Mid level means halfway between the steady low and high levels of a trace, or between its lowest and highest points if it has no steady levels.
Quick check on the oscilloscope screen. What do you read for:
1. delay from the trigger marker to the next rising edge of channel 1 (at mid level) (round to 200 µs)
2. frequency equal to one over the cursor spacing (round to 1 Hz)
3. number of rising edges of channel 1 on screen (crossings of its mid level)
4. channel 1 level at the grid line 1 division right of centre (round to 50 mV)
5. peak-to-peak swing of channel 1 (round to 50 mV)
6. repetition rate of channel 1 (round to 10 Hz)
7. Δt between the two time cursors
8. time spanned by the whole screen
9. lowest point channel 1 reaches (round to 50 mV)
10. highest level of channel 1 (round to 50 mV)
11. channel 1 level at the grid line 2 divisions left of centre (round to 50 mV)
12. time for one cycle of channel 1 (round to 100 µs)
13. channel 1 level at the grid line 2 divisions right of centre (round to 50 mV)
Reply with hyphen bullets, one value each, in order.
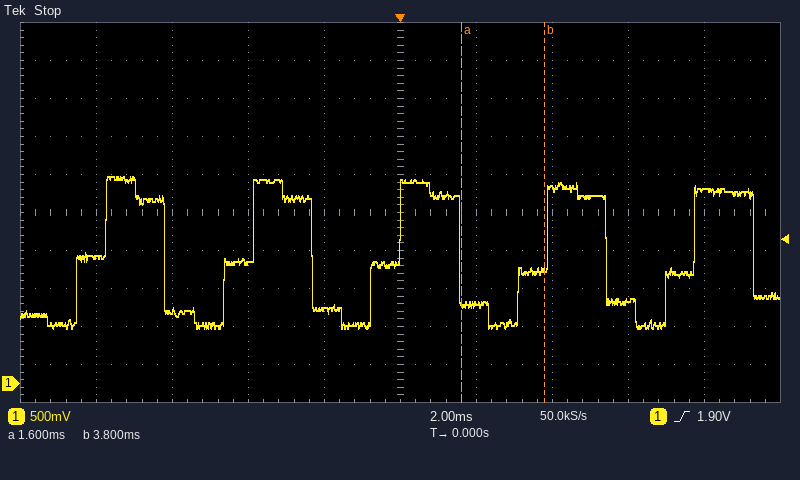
- 3.8 ms
- 455 Hz
- 5
- 1.05 V
- 2.00 V
- 260 Hz
- 2.2 ms
- 20 ms
- 700 mV
- 2.70 V
- 1.60 V
- 3.9 ms
- 2.55 V
